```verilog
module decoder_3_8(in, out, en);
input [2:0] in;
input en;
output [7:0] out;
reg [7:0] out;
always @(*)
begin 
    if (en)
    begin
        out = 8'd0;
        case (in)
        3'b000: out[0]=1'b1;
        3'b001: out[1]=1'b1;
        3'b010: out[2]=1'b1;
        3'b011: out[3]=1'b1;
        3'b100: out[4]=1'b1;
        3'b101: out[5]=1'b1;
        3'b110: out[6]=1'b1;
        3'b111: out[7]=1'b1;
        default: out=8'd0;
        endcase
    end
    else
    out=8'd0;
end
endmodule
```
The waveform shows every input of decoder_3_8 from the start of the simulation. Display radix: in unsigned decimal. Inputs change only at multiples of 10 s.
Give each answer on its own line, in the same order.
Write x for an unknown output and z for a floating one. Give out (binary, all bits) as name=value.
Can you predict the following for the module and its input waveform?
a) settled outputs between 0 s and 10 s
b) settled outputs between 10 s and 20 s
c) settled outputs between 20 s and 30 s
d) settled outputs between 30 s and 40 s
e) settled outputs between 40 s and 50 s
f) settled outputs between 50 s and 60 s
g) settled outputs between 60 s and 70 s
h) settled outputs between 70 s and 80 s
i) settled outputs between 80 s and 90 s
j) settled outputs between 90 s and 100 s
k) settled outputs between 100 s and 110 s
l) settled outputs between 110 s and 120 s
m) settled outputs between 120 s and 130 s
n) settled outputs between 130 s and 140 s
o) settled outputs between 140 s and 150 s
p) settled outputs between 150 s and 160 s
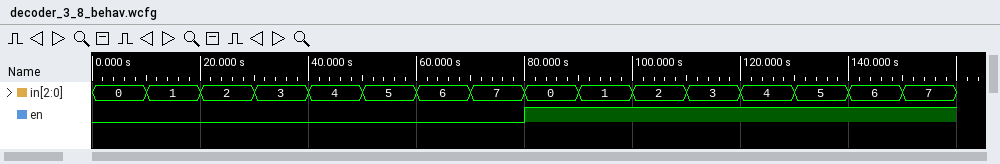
out=00000000
out=00000000
out=00000000
out=00000000
out=00000000
out=00000000
out=00000000
out=00000000
out=00000001
out=00000010
out=00000100
out=00001000
out=00010000
out=00100000
out=01000000
out=10000000
